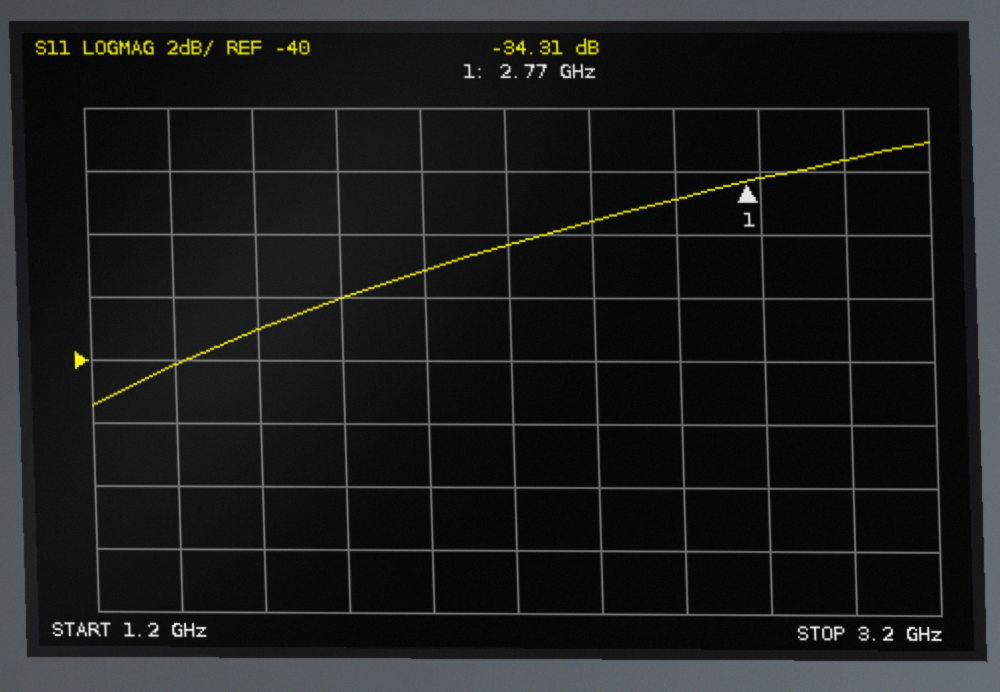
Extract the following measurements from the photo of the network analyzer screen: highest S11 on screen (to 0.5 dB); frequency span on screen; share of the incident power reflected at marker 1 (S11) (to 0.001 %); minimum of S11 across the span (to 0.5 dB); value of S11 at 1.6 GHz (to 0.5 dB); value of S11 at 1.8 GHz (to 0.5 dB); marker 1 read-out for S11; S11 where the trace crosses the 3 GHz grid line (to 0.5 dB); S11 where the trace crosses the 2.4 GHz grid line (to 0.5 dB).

-33.0 dB
2 GHz
0.037 %
-41.5 dB
-39.0 dB
-38.0 dB
-34.31 dB
-33.5 dB
-35.5 dB
